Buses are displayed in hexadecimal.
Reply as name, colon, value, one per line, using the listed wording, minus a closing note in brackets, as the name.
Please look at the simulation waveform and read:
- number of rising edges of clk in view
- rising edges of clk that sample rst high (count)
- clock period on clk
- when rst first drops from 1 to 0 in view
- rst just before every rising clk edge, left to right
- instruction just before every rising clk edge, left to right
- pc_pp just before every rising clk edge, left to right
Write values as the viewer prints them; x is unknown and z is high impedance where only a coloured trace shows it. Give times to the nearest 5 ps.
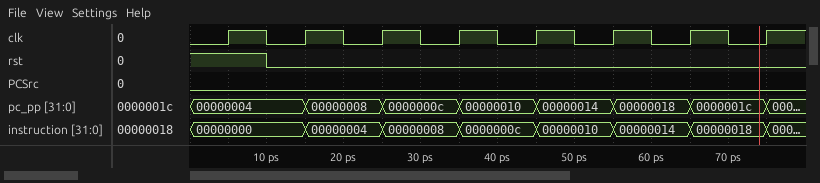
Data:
number of rising edges of clk in view: 8
rising edges of clk that sample rst high: 1
clock period on clk: 10 ps
when rst first drops from 1 to 0 in view: 10 ps
rst just before every rising clk edge, left to right: 1 0 0 0 0 0 0 0
instruction just before every rising clk edge, left to right: 00000000, 00000000, 00000004, 00000008, 0000000c, 00000010, 00000014, 00000018
pc_pp just before every rising clk edge, left to right: 00000004, 00000004, 00000008, 0000000c, 00000010, 00000014, 00000018, 0000001c
